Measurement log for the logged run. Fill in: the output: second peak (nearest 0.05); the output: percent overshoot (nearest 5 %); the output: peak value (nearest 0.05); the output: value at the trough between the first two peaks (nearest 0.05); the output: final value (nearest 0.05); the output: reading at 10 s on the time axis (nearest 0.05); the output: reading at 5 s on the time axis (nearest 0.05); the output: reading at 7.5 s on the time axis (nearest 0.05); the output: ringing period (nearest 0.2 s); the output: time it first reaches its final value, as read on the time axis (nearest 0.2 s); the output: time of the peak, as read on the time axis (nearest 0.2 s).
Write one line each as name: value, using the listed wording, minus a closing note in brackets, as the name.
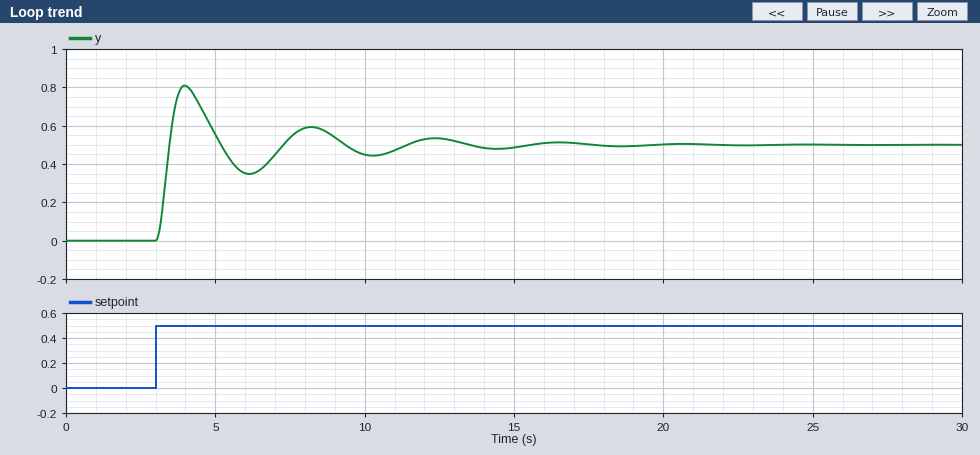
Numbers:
the output: second peak: 0.60
the output: percent overshoot: 60 %
the output: peak value: 0.80
the output: value at the trough between the first two peaks: 0.35
the output: final value: 0.50
the output: reading at 10 s on the time axis: 0.45
the output: reading at 5 s on the time axis: 0.55
the output: reading at 7.5 s on the time axis: 0.55
the output: ringing period: 4.2 s
the output: time it first reaches its final value, as read on the time axis: 3.4 s
the output: time of the peak, as read on the time axis: 4.0 s
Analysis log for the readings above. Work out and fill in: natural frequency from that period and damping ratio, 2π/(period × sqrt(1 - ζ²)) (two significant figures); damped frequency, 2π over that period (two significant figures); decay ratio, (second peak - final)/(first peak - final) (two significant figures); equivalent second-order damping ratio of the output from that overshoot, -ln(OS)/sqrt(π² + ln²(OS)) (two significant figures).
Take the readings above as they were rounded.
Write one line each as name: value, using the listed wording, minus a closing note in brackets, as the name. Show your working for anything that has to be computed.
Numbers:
natural frequency from that period and damping ratio, 2π/(period × sqrt(1 - ζ²)): 2π / (4.2 × sqrt(1 - 0.16²)) = 1.5 rad/s
damped frequency, 2π over that period: 2π / 4.2 = 1.5 rad/s
decay ratio, (second peak - final)/(first peak - final): (0.6 - 0.5) / (0.8 - 0.5) = 0.33
equivalent second-order damping ratio of the output from that overshoot, -ln(OS)/sqrt(π² + ln²(OS)): ln(0.6) = -0.511; 0.511 / sqrt(9.870 + 0.261) = 0.16
